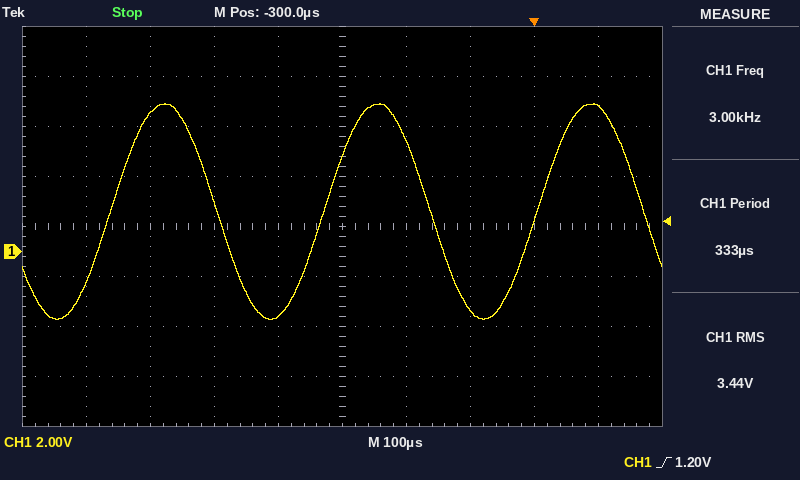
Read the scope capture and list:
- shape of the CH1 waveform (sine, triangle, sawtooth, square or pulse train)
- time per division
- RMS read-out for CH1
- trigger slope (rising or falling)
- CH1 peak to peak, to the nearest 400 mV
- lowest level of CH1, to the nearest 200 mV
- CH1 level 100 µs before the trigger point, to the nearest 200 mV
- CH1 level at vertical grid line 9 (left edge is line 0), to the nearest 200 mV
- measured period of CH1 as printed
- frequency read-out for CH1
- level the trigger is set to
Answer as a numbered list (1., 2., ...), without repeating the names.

1. sine
2. 100 µs
3. 3.44 V
4. rising
5. 8.8 V
6. -2.8 V
7. -2.4 V
8. 5.8 V
9. 333 µs
10. 3.00 kHz
11. 1.20 V
